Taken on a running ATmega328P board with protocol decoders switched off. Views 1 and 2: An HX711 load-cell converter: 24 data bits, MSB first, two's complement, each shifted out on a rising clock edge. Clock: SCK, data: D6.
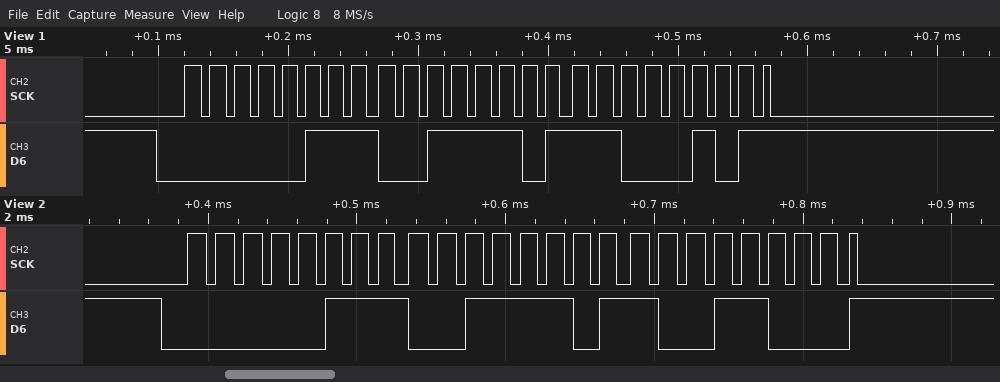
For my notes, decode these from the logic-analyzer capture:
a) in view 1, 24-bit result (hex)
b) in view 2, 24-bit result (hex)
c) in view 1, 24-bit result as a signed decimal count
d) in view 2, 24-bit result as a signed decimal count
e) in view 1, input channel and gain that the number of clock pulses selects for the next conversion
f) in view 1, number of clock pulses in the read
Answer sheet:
0x073DC5
0x073D98
474565
474520
channel A, gain 128
25
